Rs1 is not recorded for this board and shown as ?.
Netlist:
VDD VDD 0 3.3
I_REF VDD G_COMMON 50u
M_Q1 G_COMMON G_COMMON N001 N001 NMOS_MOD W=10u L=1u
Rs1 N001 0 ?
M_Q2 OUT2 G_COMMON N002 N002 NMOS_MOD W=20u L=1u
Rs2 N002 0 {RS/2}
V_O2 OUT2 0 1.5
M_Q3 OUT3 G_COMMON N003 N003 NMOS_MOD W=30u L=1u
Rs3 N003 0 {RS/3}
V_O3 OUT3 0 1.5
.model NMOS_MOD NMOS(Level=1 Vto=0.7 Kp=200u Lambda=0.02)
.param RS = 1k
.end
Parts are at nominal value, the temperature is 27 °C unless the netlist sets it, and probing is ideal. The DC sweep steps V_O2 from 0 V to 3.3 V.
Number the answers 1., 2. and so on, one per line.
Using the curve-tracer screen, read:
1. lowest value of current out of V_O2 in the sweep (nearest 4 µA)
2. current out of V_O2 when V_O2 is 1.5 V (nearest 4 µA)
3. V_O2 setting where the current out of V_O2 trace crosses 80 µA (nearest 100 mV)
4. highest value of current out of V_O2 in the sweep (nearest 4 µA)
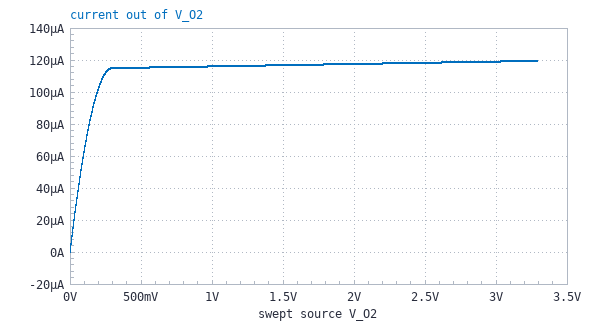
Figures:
1. 0 A
2. 116 µA
3. 100 mV
4. 120 µA
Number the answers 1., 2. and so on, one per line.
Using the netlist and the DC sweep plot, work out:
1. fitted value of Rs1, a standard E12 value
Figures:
1. 1.5 kΩ
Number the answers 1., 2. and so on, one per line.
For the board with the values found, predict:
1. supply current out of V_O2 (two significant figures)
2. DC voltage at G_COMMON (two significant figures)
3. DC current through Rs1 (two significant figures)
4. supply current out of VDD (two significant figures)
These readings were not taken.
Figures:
1. 120 µA
2. 1.0 V
3. 50 µA
4. 50 µA
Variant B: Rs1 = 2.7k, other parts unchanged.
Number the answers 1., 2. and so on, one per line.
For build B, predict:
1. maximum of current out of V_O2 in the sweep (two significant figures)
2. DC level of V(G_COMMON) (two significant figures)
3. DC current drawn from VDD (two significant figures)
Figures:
1. 160 µA
2. 1.1 V
3. 50 µA
